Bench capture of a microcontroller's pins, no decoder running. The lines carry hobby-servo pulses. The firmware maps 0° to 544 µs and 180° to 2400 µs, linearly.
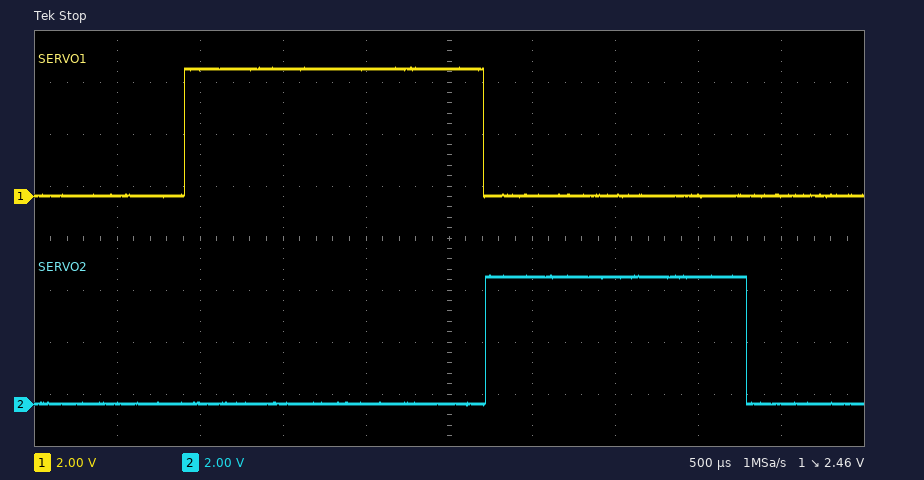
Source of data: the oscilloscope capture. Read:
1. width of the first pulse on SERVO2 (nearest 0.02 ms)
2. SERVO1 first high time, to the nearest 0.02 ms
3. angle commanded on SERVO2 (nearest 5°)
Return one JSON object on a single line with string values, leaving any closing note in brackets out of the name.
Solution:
{"width of the first pulse on SERVO2": "1.58 ms", "SERVO1 first high time, to the nearest 0.02 ms": "1.80 ms", "angle commanded on SERVO2": "100°"}
